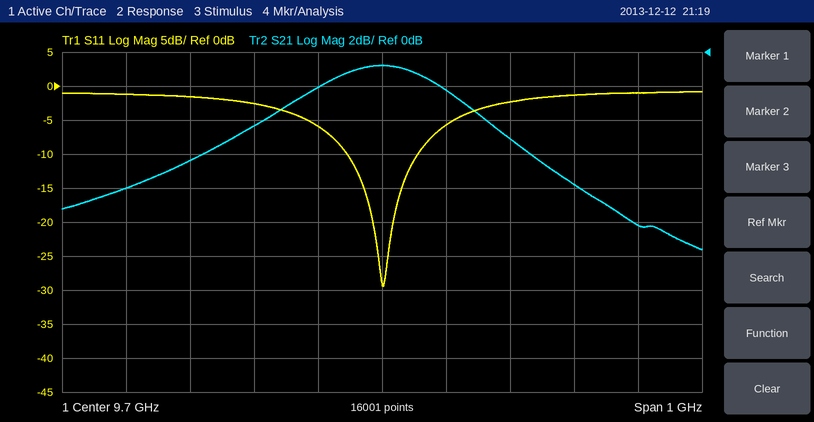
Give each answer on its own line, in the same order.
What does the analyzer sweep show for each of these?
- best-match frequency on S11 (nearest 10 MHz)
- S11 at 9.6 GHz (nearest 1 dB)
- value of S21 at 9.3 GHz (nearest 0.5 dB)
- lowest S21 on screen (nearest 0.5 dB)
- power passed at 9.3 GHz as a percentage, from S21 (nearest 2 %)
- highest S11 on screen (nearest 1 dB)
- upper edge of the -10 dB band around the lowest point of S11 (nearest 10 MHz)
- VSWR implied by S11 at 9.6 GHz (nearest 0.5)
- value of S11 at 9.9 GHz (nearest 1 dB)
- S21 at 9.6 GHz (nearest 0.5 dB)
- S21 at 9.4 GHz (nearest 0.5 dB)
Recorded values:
9.70 GHz
-6 dB
-8.0 dB
-11.5 dB
16 %
-1 dB
9.76 GHz
3.0
-2 dB
-2.0 dB
-6.5 dB
